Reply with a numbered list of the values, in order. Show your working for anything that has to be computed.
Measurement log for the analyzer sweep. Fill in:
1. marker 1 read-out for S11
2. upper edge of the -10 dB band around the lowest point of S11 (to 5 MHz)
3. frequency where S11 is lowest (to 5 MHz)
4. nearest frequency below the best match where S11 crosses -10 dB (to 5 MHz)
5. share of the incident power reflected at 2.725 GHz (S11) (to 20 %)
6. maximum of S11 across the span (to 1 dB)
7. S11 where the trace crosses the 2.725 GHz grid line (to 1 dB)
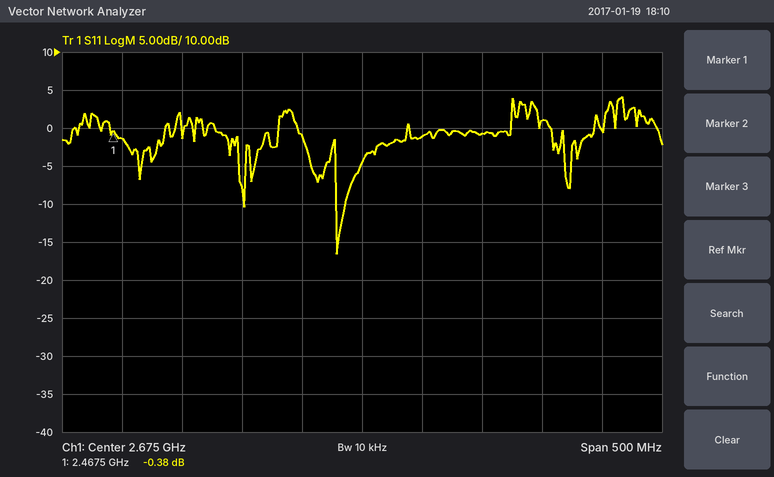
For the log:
1. -0.38 dB
2. 2.660 GHz
3. 2.655 GHz
4. 2.655 GHz
5. 10^(-1/10) ≈ 79.4 %, so 80 % to the nearest 20 %
6. 4 dB
7. -1 dB
